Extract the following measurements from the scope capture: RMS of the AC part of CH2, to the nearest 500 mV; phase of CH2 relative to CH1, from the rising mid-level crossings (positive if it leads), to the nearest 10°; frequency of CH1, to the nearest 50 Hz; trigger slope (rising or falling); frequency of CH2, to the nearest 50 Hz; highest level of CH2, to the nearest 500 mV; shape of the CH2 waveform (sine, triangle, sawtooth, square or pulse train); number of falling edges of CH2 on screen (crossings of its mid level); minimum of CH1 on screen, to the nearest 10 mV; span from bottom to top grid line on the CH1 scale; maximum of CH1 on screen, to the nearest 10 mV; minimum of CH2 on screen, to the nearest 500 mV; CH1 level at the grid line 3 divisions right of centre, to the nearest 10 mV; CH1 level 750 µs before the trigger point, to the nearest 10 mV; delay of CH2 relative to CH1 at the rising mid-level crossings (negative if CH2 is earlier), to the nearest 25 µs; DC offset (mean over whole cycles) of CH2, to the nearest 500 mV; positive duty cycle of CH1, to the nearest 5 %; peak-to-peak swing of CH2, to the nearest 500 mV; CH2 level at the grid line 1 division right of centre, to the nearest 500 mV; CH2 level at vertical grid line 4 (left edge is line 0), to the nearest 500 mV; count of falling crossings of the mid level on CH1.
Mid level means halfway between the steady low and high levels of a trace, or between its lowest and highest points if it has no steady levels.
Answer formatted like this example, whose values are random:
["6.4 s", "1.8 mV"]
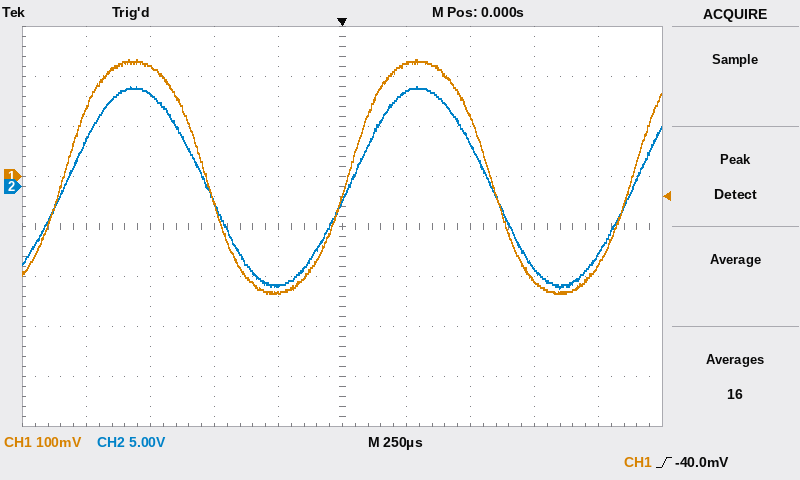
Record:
["7.0 V", "0°", "900 Hz", "rising", "900 Hz", "10.0 V", "sine", "2", "-230 mV", "800 mV", "230 mV", "-10.0 V", "-210 mV", "220 mV", "0 µs", "0.0 V", "50 %", "20.0 V", "9.5 V", "-10.0 V", "2"]
